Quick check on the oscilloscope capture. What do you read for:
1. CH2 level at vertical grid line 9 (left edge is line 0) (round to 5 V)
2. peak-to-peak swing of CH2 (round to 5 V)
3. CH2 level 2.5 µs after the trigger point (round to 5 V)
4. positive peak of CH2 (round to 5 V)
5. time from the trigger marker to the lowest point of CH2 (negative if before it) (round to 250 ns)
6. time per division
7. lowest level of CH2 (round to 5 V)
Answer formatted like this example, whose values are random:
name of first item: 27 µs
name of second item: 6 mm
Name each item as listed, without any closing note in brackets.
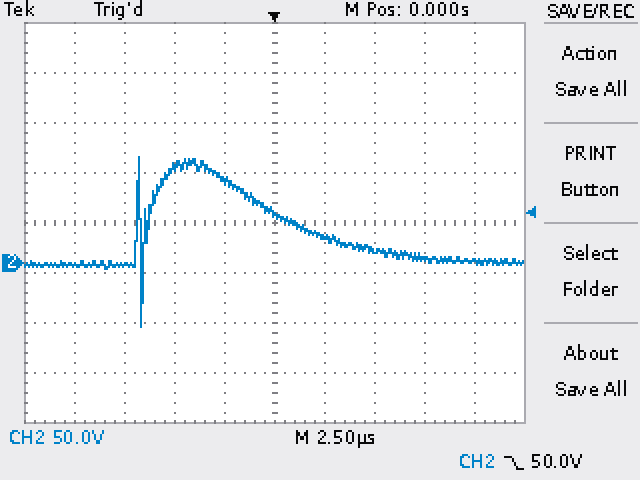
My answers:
CH2 level at vertical grid line 9 (left edge is line 0): 0 V
peak-to-peak swing of CH2: 170 V
CH2 level 2.5 µs after the trigger point: 25 V
positive peak of CH2: 105 V
time from the trigger marker to the lowest point of CH2 (negative if before it): -6.75 µs
time per division: 2.5 µs
lowest level of CH2: -65 V
